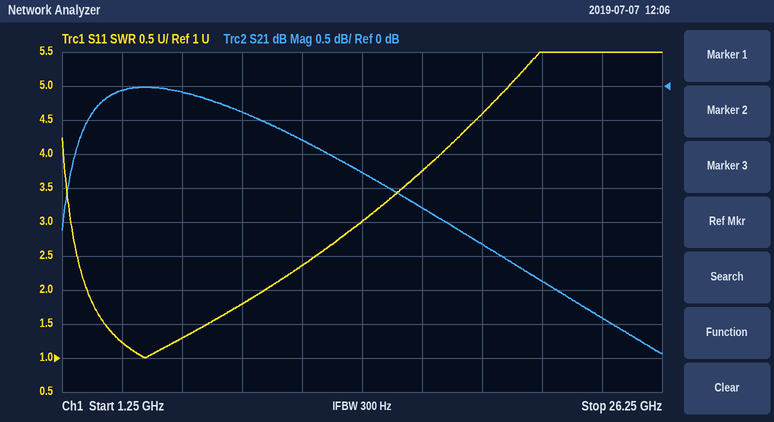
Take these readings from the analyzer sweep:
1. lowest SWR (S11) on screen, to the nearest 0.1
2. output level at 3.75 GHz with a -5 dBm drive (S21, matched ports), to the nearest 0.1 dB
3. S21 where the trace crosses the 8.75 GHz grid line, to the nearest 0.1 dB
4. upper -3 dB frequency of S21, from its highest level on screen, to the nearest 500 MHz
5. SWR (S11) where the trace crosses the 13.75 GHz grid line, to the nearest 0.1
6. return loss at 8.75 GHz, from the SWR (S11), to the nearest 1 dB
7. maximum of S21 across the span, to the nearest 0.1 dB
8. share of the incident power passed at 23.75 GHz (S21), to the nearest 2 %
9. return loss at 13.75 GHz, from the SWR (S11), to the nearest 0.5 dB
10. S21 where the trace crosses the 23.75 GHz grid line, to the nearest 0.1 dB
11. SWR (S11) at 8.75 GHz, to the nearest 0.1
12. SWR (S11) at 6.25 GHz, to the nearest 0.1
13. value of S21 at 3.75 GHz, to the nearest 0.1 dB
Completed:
1.0
-5.1 dBm
-0.4 dB
22.0 GHz
3.0
11 dB
0.0 dB
46 %
6.0 dB
-3.4 dB
1.8
1.3
-0.1 dB
